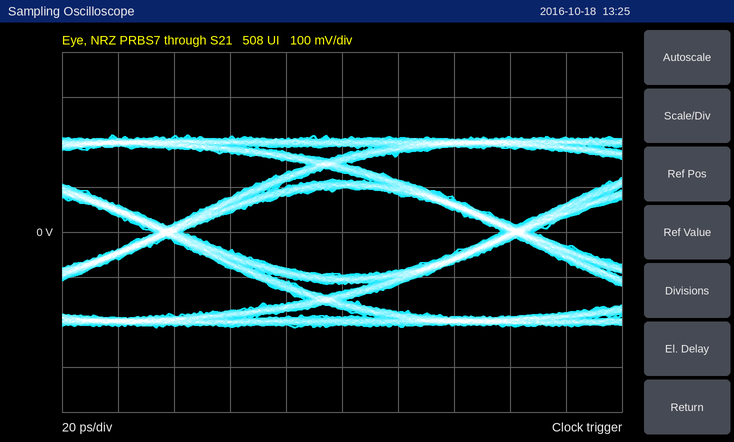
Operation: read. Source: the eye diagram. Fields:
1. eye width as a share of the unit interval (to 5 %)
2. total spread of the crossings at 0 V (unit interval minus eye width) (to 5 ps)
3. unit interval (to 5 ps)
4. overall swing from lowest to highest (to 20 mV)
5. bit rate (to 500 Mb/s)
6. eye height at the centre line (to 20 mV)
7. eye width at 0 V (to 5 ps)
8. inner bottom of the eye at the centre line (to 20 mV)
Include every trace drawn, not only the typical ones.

90 %
10 ps
125 ps
420 mV
8.0 Gb/s
200 mV
115 ps
-100 mV
